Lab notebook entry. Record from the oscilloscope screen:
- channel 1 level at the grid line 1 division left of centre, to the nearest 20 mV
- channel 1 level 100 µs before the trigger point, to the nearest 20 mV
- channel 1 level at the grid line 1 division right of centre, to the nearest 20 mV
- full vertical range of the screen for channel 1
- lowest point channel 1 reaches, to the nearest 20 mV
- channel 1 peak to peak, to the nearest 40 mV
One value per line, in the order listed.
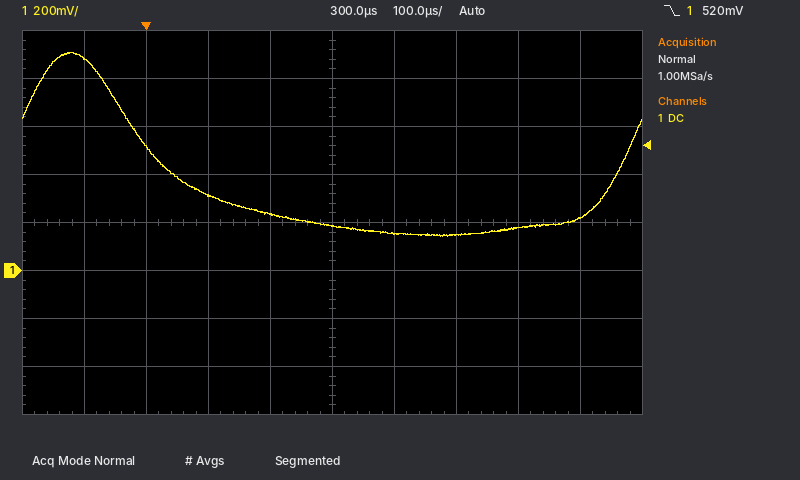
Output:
240 mV
880 mV
160 mV
1.6 V
140 mV
760 mV
